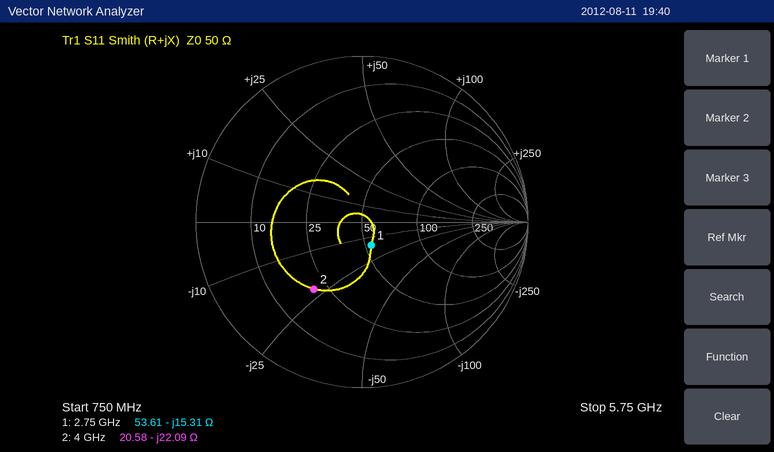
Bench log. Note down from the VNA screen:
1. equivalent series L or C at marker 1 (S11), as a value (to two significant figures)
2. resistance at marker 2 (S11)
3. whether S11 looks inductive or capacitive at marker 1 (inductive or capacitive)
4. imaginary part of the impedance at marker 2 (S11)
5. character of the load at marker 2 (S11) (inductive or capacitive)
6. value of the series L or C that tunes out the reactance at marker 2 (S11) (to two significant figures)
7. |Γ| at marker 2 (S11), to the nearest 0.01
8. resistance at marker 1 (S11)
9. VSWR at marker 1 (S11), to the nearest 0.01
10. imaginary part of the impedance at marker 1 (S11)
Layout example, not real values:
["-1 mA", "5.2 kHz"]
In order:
["3.8 pF", "20.58 Ω", "capacitive", "-22.09 Ω", "capacitive", "880 pH", "0.50", "53.61 Ω", "1.35", "-15.31 Ω"]
